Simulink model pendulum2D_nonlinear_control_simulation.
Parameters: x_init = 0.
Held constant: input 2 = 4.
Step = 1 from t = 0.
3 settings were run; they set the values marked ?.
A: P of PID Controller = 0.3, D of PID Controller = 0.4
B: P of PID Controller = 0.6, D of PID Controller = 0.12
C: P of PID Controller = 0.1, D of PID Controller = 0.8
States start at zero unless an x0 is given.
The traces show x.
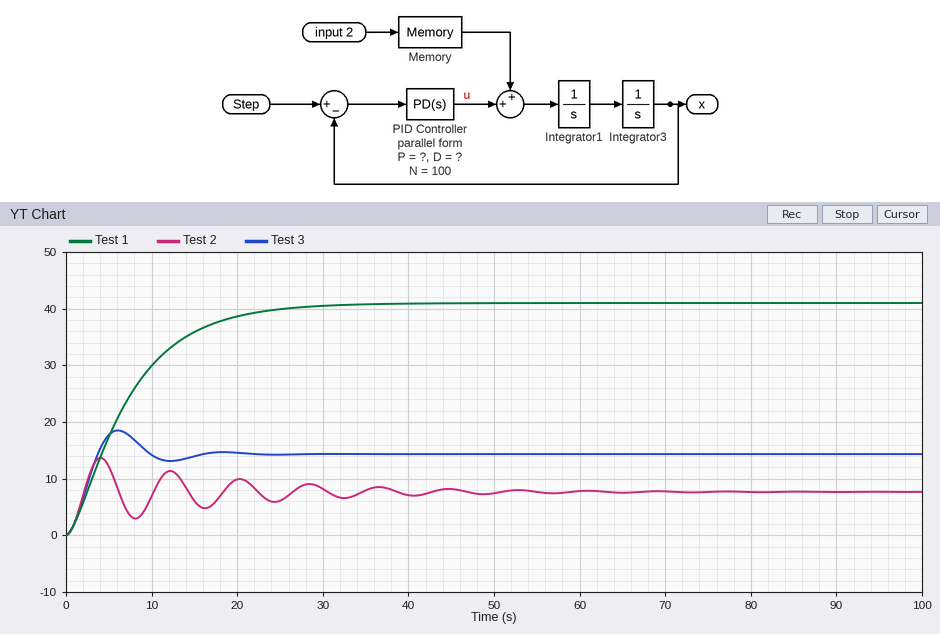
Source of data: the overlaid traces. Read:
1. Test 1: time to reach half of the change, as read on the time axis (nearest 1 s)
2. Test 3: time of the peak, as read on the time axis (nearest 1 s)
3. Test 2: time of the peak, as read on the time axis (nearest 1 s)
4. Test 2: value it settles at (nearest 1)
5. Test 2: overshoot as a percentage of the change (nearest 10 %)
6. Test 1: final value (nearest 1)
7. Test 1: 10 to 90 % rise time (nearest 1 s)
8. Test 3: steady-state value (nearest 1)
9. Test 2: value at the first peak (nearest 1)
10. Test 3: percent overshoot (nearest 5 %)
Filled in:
6 s
6 s
4 s
8
80 %
41
15 s
14
14
30 %
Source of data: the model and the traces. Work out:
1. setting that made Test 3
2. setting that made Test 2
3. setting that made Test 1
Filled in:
A
B
C
